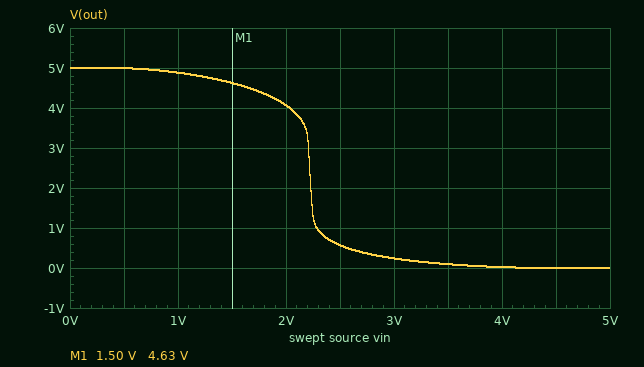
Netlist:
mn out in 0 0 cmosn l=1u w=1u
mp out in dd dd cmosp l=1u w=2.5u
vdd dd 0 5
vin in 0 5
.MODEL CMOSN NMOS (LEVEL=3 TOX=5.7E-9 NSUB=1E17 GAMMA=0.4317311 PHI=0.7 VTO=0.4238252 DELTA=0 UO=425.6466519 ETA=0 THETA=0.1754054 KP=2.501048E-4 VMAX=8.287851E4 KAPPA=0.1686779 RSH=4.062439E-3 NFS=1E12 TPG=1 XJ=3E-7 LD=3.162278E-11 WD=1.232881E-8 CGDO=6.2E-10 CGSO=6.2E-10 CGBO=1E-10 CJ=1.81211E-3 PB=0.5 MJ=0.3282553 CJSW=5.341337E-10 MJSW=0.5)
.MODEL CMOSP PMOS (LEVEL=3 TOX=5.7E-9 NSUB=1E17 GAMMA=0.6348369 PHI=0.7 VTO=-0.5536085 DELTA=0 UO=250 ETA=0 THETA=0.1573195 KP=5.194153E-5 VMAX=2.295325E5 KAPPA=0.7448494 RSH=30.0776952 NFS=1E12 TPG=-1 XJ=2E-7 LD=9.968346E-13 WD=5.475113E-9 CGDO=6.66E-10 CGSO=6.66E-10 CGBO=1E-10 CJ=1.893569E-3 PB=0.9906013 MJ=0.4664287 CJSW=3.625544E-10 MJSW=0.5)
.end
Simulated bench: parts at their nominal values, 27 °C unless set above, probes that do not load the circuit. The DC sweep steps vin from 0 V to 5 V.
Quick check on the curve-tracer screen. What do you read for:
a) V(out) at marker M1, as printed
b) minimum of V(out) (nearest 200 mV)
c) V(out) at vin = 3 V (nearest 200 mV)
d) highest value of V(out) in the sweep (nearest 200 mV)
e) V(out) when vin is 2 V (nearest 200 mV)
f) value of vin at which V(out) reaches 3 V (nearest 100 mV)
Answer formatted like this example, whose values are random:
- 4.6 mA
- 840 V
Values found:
- 4.63 V
- 0 V
- 200 mV
- 5.0 V
- 4.0 V
- 2.2 V
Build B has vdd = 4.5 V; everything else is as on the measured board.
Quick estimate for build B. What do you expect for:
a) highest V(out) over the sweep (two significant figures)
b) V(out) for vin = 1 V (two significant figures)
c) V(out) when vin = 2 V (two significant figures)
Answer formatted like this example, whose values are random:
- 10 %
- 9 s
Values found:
- 4.5 V
- 4.4 V
- 1.5 V
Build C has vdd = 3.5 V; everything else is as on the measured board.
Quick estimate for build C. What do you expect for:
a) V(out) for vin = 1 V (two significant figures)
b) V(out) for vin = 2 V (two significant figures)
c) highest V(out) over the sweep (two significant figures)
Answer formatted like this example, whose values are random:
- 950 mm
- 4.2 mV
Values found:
- 3.3 V
- 160 mV
- 3.5 V
